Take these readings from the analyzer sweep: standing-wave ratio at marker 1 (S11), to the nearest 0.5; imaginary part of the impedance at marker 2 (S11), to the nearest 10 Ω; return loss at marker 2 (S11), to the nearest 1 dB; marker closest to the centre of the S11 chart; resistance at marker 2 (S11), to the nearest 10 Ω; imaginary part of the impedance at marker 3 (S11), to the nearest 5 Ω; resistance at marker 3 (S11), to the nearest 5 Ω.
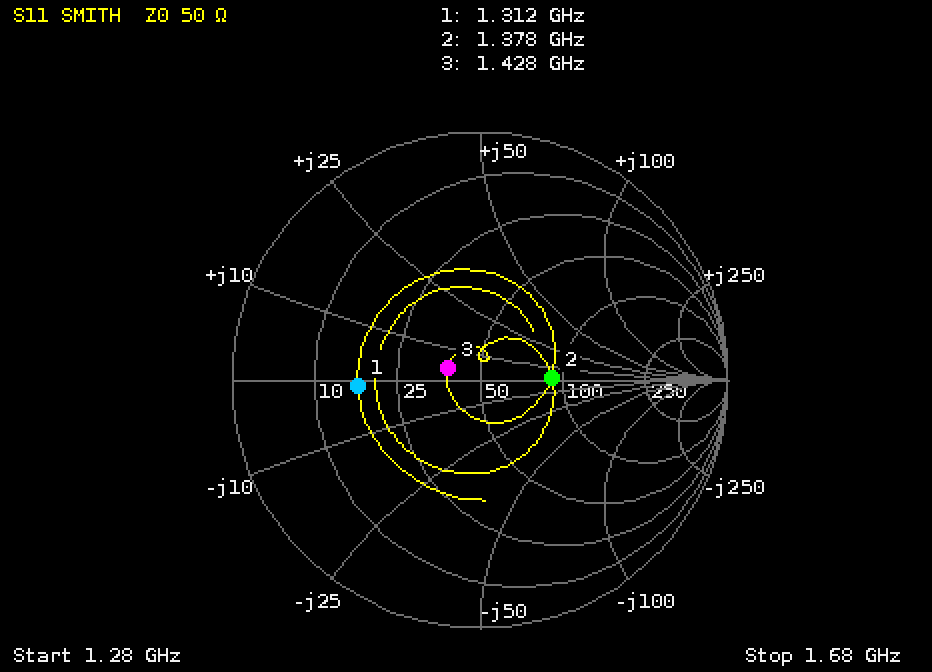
3.0
0 Ω
11 dB
marker 3
90 Ω
+5 Ω
40 Ω
